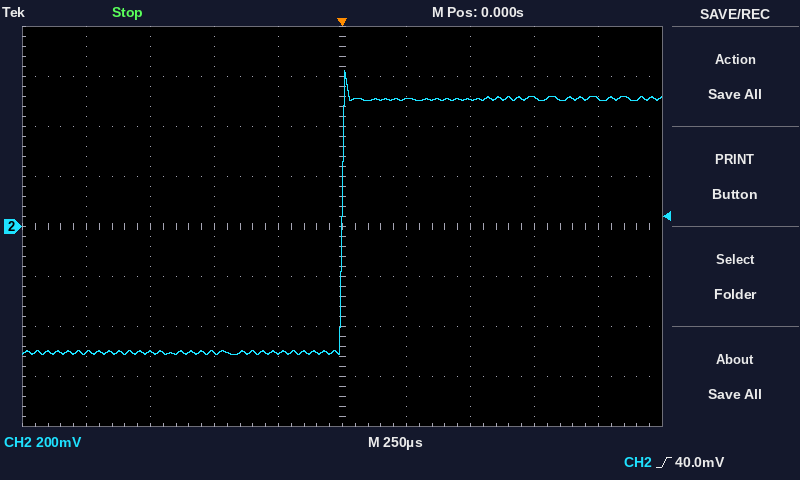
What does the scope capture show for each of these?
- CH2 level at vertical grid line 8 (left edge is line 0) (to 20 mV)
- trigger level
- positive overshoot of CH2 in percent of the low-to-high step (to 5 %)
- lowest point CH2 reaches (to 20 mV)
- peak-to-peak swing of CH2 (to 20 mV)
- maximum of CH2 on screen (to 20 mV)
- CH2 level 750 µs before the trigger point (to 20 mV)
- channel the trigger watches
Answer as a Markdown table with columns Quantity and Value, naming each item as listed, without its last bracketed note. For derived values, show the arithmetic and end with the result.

| Quantity | Value |
|---|---|
| CH2 level at vertical grid line 8 (left edge is line 0) | 520 mV |
| trigger level | 40.0 mV |
| positive overshoot of CH2 in percent of the low-to-high step | 10 % |
| lowest point CH2 reaches | -520 mV |
| peak-to-peak swing of CH2 | 620 mV − (-520 mV) = 1.14 V |
| maximum of CH2 on screen | 620 mV |
| CH2 level 750 µs before the trigger point | -500 mV |
| channel the trigger watches | CH2 |
